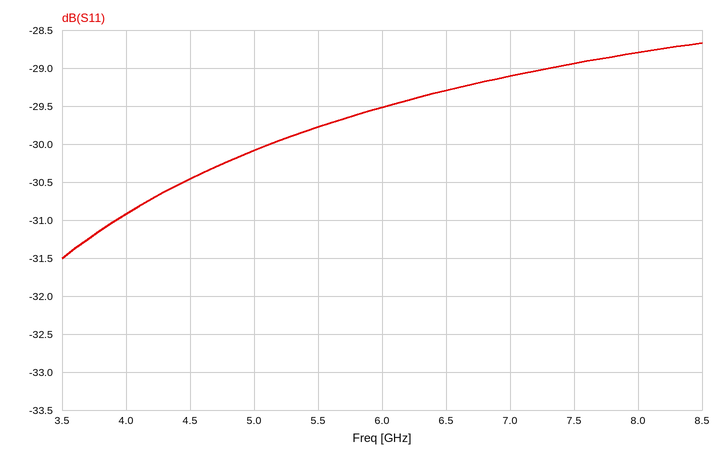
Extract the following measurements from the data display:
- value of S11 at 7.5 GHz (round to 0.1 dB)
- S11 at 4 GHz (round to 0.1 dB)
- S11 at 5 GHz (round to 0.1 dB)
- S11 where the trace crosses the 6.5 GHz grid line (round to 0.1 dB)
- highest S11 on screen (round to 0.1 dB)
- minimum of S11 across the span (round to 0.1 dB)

-28.9 dB
-30.9 dB
-30.1 dB
-29.3 dB
-28.7 dB
-31.5 dB
